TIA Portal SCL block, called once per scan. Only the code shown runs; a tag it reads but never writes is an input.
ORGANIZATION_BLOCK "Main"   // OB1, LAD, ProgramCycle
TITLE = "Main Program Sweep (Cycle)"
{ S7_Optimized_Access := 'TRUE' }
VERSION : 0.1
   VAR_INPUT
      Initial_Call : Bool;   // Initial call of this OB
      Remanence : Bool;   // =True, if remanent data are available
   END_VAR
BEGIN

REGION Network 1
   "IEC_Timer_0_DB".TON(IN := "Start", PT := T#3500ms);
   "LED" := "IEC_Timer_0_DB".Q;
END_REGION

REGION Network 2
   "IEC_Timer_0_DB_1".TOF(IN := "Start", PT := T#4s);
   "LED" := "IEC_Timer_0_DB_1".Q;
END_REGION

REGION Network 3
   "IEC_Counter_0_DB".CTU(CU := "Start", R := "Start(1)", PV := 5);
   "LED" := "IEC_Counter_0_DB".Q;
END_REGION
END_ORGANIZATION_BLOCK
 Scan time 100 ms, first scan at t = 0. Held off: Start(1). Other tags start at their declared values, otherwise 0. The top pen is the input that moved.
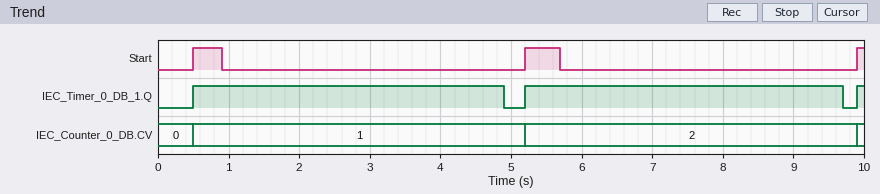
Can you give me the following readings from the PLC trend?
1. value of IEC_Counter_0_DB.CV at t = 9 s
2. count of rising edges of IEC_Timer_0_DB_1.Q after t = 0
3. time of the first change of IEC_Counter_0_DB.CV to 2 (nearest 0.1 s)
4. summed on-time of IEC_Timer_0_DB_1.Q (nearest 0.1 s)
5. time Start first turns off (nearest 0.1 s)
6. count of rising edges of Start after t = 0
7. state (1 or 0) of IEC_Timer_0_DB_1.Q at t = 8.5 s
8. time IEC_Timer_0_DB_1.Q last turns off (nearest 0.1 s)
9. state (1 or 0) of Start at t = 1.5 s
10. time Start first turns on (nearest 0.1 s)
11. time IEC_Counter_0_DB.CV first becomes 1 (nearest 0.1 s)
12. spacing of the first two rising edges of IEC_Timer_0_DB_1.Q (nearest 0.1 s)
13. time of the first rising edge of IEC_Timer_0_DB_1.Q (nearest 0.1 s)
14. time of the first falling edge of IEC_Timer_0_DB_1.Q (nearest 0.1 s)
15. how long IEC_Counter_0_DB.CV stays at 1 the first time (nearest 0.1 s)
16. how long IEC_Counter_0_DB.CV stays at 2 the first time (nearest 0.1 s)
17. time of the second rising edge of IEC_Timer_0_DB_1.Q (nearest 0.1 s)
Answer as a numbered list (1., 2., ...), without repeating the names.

1. 2
2. 3
3. 5.2 s
4. 9.0 s
5. 0.9 s
6. 3
7. 1
8. 9.7 s
9. 0
10. 0.5 s
11. 0.5 s
12. 4.7 s
13. 0.5 s
14. 4.9 s
15. 4.7 s
16. 4.7 s
17. 5.2 s
